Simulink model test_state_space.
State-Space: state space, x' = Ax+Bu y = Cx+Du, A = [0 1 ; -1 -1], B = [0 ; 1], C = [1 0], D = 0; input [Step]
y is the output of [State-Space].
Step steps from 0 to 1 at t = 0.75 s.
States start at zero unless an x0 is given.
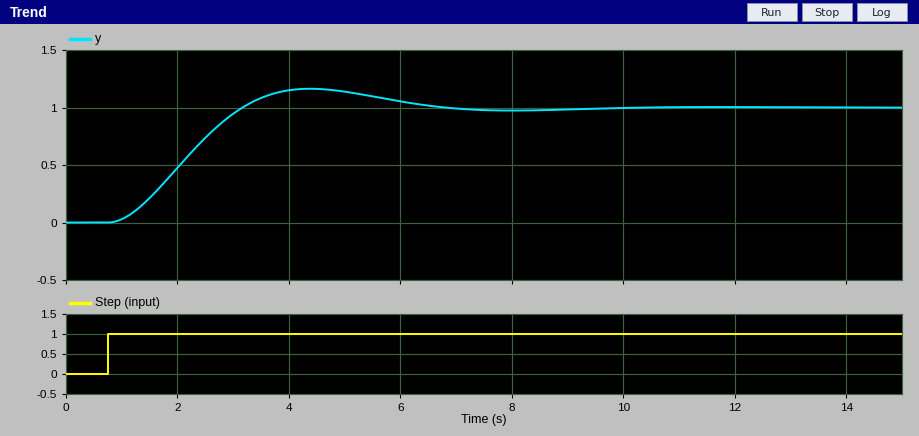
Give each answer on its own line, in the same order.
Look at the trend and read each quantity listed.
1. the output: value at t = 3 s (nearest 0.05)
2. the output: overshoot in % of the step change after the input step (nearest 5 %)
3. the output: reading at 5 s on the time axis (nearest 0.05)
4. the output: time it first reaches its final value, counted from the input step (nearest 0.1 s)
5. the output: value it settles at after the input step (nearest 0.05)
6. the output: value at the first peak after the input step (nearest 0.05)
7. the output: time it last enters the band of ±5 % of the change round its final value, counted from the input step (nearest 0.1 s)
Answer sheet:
0.95
15 %
1.15
2.4 s
1.00
1.15
5.3 s
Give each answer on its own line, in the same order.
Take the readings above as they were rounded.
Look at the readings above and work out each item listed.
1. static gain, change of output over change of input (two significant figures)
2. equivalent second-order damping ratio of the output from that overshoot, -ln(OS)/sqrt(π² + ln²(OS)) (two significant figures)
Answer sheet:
1.0
0.52
